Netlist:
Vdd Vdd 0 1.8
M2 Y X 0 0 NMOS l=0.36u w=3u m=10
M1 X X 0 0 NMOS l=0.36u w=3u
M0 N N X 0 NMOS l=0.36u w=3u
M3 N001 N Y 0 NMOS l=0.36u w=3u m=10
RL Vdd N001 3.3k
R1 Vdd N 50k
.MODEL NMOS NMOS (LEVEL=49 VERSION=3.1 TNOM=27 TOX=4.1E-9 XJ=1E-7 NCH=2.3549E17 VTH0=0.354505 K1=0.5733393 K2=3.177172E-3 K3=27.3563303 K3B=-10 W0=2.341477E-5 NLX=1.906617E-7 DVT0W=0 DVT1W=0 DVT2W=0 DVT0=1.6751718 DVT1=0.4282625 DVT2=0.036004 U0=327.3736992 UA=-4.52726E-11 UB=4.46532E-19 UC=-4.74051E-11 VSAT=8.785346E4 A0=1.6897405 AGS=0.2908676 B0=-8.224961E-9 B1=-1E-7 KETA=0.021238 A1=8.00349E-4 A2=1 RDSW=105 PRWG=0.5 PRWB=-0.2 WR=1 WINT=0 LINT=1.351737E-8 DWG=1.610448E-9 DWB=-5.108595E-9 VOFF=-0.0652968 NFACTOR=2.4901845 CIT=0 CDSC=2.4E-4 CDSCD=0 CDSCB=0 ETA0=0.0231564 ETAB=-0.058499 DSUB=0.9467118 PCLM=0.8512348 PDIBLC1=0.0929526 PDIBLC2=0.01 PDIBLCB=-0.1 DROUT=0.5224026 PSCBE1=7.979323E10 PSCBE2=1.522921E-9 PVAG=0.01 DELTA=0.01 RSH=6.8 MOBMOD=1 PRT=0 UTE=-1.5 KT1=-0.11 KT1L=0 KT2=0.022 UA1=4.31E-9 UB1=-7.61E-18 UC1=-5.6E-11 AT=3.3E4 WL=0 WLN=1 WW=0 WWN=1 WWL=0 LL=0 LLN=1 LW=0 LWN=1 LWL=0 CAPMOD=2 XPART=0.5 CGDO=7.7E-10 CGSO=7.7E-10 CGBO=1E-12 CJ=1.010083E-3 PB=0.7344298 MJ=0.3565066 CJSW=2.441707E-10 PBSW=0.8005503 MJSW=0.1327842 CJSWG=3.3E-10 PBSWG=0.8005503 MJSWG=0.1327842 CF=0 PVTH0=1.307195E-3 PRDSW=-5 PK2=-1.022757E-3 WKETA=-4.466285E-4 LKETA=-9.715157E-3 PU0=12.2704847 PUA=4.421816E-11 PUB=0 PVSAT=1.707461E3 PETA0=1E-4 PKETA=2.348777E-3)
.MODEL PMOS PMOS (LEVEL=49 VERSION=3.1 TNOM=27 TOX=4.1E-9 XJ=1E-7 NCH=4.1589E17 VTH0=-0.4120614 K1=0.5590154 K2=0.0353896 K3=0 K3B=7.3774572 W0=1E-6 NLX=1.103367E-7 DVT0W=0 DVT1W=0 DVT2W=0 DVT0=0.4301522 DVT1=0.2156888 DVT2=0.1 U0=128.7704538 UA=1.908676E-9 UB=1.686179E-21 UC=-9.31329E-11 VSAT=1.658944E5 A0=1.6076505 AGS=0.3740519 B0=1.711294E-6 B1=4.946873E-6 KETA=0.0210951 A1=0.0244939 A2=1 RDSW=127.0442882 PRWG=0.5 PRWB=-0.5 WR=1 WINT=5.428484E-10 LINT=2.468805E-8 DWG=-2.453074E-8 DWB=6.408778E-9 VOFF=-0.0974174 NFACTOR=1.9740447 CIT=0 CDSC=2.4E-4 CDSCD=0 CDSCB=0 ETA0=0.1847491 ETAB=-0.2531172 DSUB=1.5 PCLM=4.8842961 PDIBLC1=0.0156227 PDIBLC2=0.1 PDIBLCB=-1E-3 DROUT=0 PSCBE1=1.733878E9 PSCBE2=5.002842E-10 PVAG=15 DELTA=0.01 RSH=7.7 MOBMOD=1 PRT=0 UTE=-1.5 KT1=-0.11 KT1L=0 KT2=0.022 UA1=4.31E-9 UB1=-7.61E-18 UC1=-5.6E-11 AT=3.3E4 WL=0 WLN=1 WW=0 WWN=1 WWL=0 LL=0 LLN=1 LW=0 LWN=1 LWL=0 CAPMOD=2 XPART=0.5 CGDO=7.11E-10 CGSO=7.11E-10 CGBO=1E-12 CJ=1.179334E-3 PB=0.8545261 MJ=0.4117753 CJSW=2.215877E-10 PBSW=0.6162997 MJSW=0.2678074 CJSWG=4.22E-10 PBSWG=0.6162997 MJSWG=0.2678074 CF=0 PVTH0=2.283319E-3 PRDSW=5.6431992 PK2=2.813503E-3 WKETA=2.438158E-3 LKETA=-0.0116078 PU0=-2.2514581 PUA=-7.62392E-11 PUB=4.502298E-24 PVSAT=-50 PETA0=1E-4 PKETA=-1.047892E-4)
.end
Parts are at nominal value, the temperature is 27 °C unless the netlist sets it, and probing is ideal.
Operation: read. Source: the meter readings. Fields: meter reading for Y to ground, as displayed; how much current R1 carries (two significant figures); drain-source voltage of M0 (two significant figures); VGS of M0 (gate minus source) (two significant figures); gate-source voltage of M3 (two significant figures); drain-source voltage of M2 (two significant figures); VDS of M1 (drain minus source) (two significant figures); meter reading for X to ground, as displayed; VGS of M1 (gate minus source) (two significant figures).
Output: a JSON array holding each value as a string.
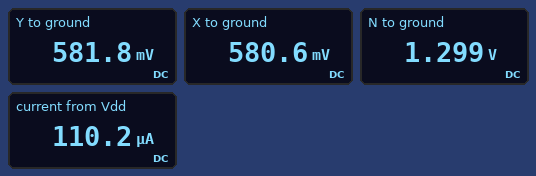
["581.8 mV", "10 µA", "720 mV", "720 mV", "720 mV", "580 mV", "580 mV", "580.6 mV", "580 mV"]
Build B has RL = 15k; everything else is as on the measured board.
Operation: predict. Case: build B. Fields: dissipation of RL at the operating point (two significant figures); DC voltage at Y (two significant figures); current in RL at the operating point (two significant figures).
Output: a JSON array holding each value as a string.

["140 µW", "350 mV", "96 µA"]
